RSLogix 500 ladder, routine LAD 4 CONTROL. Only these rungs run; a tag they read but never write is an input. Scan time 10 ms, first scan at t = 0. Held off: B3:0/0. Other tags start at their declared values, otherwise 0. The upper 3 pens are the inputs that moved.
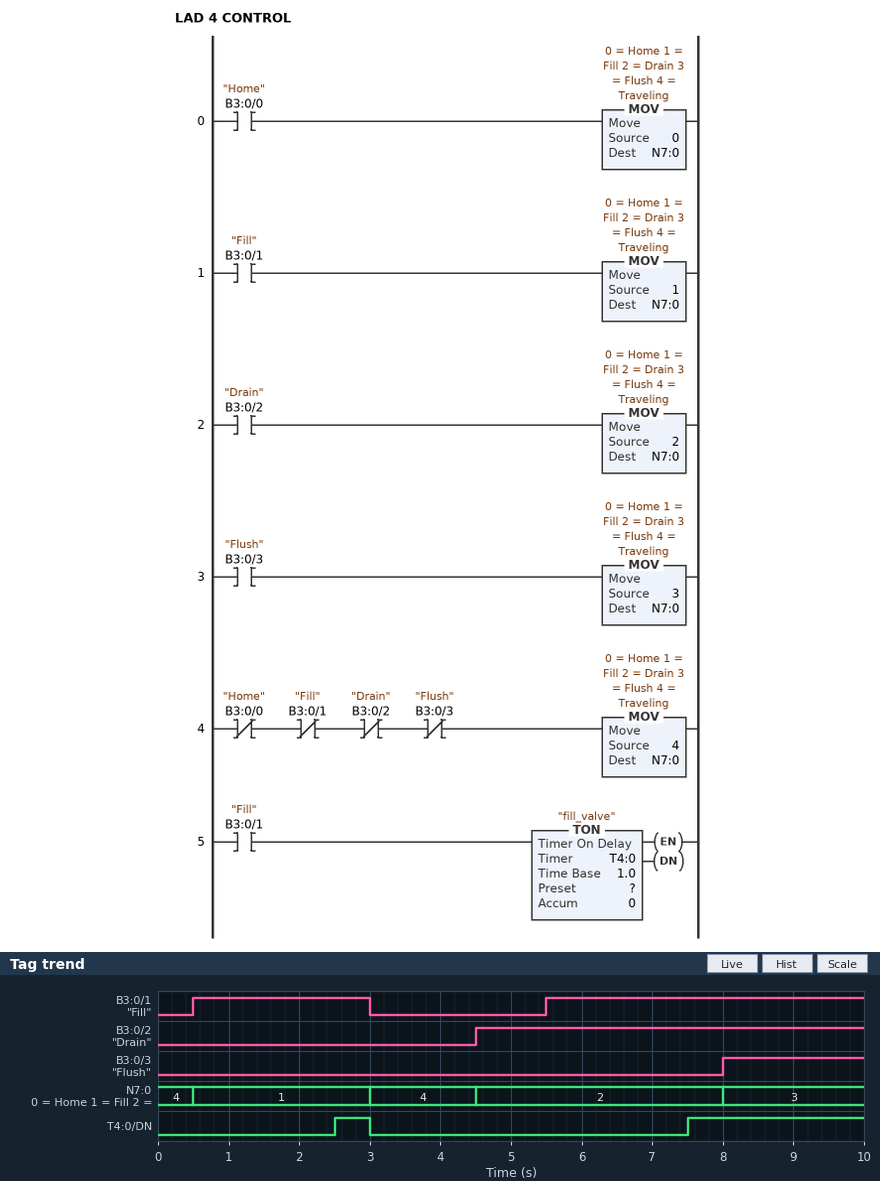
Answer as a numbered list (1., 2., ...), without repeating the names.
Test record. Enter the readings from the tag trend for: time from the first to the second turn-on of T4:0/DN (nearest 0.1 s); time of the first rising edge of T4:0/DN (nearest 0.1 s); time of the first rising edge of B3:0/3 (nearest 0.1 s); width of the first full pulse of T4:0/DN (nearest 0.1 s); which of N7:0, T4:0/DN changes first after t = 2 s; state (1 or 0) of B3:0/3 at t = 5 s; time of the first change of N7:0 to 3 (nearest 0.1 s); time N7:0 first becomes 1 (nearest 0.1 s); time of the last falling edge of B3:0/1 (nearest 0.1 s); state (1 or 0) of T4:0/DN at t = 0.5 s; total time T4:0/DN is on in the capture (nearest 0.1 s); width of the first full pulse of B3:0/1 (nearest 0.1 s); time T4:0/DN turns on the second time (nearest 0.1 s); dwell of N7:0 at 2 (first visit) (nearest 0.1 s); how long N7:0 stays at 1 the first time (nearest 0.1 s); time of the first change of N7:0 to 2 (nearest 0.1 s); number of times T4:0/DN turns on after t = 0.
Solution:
1. 5.0 s
2. 2.5 s
3. 8.0 s
4. 0.5 s
5. T4:0/DN
6. 0
7. 8.0 s
8. 0.5 s
9. 3.0 s
10. 0
11. 3.0 s
12. 2.5 s
13. 7.5 s
14. 3.5 s
15. 2.5 s
16. 4.5 s
17. 2
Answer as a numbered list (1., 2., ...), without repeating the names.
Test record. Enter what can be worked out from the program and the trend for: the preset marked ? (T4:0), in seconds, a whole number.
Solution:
1. 2 s
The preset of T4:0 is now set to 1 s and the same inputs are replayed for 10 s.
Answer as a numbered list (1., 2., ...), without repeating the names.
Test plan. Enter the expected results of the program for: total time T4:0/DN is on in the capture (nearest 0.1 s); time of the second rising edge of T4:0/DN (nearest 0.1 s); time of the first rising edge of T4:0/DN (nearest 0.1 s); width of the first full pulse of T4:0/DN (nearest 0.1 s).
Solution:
1. 5.0 s
2. 6.5 s
3. 1.5 s
4. 1.5 s
